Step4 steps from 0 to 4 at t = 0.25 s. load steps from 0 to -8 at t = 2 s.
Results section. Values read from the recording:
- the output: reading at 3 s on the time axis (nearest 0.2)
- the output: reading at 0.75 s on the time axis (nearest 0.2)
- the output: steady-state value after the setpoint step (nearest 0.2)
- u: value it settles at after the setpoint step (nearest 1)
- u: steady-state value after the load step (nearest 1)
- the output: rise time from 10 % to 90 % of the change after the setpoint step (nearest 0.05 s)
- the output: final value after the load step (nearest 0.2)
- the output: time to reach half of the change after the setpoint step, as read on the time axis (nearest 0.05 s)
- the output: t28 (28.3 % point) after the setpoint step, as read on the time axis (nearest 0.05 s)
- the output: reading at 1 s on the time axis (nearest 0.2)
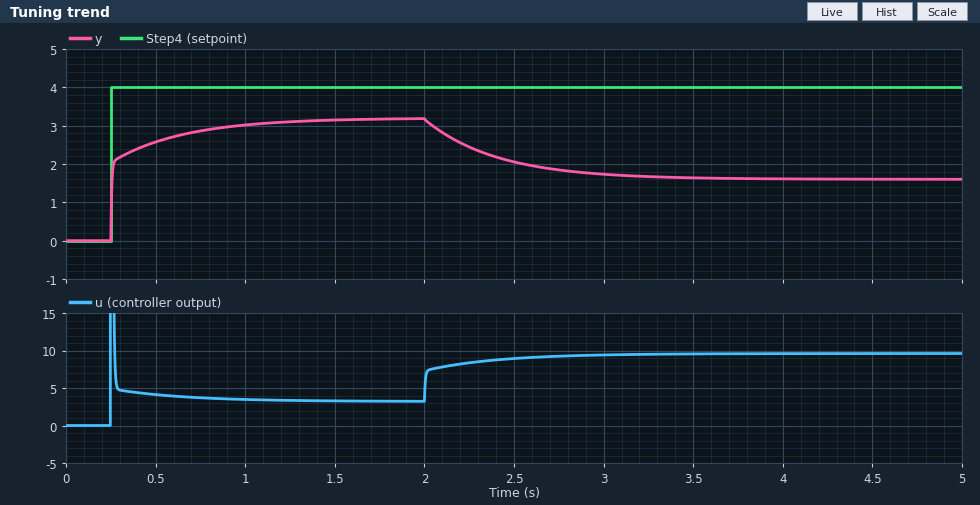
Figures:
1.8
2.8
3.2
3
10
0.50 s
1.6
0.25 s
0.25 s
3.0
